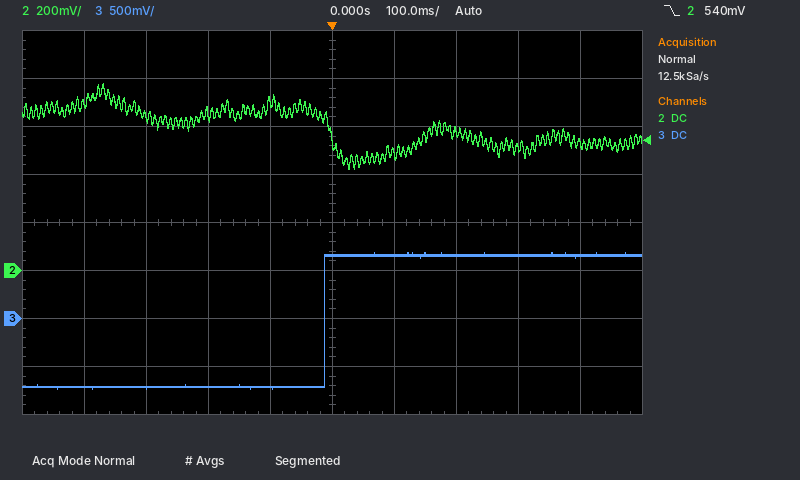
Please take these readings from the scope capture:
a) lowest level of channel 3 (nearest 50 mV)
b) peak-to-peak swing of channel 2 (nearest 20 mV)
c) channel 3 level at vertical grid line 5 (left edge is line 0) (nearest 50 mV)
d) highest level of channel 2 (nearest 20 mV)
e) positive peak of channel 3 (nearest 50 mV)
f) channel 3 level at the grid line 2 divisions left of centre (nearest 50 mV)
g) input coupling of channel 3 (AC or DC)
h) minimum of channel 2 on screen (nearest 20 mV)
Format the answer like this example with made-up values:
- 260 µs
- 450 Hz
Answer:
- -750 mV
- 360 mV
- 650 mV
- 780 mV
- 700 mV
- -700 mV
- DC
- 420 mV
